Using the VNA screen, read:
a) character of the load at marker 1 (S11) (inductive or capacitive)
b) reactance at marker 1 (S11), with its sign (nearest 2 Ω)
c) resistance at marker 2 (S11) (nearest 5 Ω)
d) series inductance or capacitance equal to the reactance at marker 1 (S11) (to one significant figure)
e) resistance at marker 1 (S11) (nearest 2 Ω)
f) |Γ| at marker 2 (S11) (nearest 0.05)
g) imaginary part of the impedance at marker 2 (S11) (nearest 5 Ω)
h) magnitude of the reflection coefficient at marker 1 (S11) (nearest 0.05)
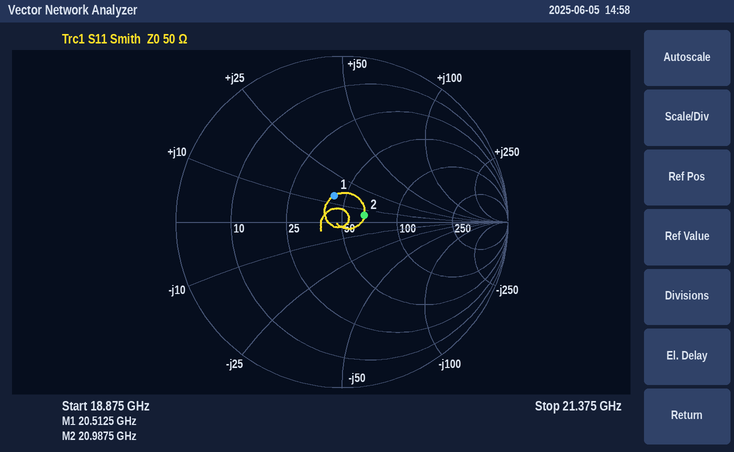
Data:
inductive
+14 Ω
65 Ω
100 pH
44 Ω
0.15
+5 Ω
0.15
